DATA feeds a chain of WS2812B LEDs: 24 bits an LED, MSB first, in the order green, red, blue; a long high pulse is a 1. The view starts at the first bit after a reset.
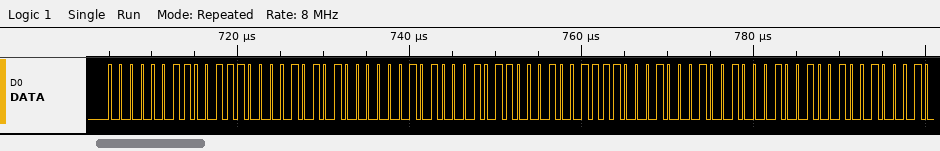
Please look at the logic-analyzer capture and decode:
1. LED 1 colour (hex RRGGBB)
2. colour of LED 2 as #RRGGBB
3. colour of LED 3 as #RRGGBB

#380354
#2C0A4F
#221149
